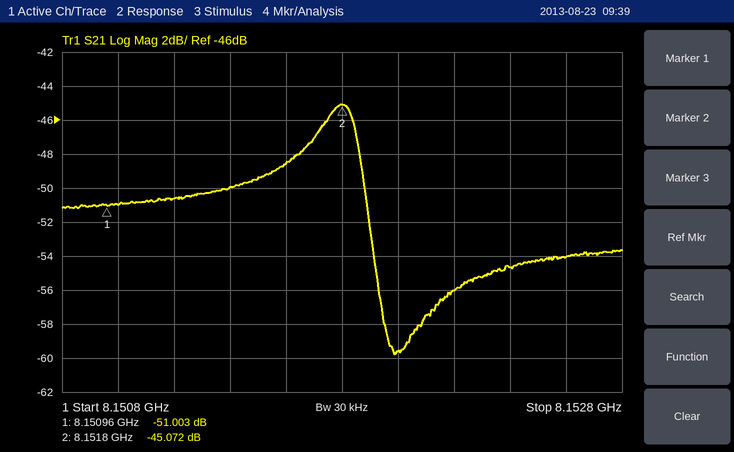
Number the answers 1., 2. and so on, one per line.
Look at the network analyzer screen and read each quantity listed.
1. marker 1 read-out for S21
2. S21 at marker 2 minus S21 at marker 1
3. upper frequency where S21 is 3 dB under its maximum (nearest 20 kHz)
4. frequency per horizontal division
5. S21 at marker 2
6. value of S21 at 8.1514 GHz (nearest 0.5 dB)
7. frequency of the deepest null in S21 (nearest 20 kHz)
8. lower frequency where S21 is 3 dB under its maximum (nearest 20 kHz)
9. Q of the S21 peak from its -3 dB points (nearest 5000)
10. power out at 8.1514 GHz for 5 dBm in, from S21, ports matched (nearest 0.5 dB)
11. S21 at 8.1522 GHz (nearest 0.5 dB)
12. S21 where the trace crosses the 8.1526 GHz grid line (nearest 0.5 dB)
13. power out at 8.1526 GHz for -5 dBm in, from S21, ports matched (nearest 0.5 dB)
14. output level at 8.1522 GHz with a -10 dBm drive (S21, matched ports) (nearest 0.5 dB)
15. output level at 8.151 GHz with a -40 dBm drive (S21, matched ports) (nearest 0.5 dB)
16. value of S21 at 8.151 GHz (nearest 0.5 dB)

1. -51.003 dB
2. 5.931 dB
3. 8.15186 GHz
4. 200 kHz
5. -45.072 dB
6. -50.0 dB
7. 8.15198 GHz
8. 8.15164 GHz
9. 35000
10. -45.0 dBm
11. -56.0 dB
12. -54.0 dB
13. -59.0 dBm
14. -66.0 dBm
15. -91.0 dBm
16. -51.0 dB
